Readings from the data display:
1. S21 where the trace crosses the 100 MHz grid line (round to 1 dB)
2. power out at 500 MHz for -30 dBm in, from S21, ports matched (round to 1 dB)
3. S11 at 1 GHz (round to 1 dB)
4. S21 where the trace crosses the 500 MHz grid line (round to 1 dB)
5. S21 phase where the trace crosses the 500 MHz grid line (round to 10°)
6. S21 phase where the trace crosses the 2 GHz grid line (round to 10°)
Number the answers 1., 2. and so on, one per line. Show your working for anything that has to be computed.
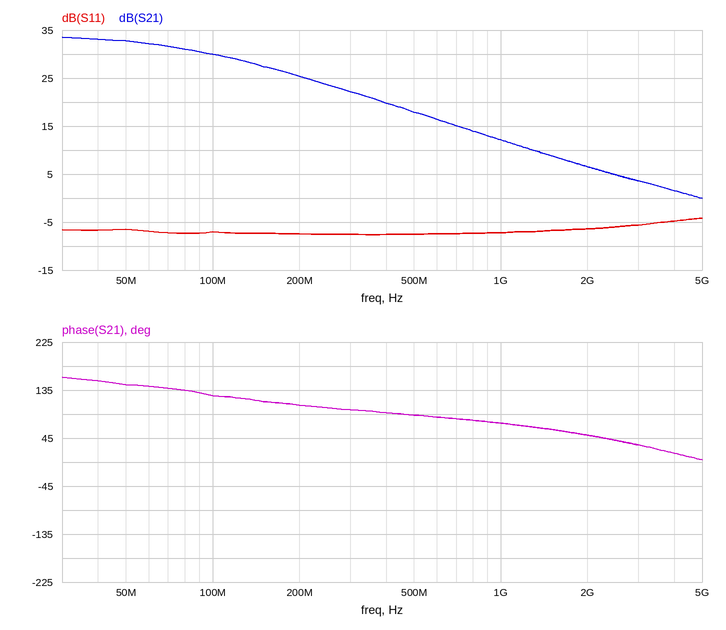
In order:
1. 30 dB
2. -30 dBm + (18 dB) = -12 dBm
3. -7 dB
4. 18 dB
5. 90°
6. 50°
